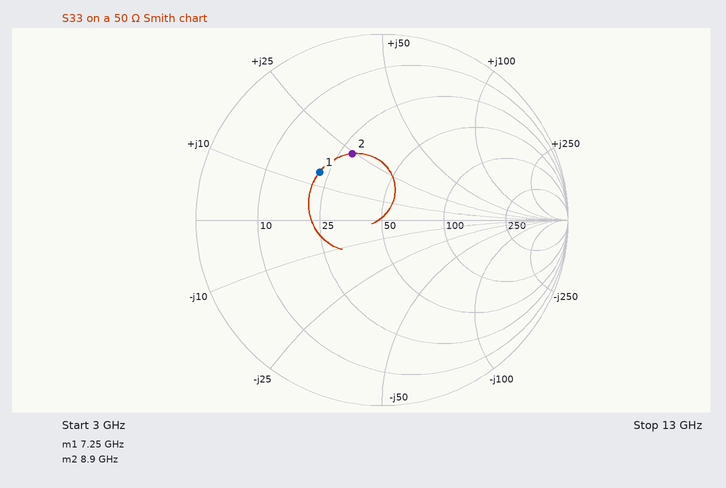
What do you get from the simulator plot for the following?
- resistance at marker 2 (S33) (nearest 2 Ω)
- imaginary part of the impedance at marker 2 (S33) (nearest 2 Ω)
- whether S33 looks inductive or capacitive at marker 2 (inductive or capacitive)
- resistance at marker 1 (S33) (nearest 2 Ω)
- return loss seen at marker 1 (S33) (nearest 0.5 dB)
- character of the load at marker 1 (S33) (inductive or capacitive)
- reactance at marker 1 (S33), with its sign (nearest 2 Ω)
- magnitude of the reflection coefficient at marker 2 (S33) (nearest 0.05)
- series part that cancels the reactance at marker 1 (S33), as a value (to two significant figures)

28 Ω
+24 Ω
inductive
22 Ω
7.5 dB
inductive
+14 Ω
0.40
1.6 pF
